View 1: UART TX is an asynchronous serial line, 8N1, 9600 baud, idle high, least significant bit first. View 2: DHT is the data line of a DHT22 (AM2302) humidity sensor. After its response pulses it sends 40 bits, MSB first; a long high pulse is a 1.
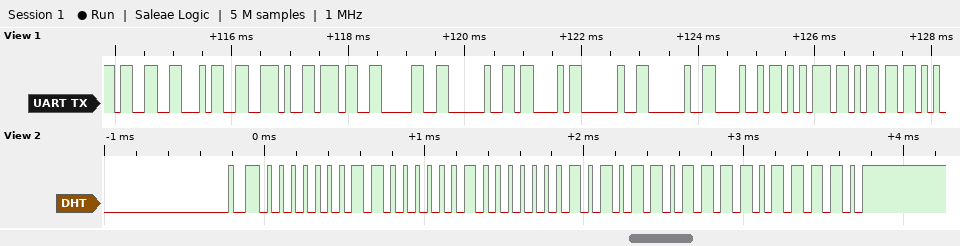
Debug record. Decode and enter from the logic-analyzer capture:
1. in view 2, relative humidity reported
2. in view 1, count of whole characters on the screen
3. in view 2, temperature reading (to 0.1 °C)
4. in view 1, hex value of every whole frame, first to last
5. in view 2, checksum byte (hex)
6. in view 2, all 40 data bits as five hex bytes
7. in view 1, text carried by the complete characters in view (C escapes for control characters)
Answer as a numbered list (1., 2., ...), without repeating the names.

1. 38.5 %
2. 12
3. 34.7 °C
4. 33 34 2E 37 30 20 43 20 20 48 75 6D
5. 0xDE
6. 01 81 01 5B DE
7. "34.70 C  Hum"
